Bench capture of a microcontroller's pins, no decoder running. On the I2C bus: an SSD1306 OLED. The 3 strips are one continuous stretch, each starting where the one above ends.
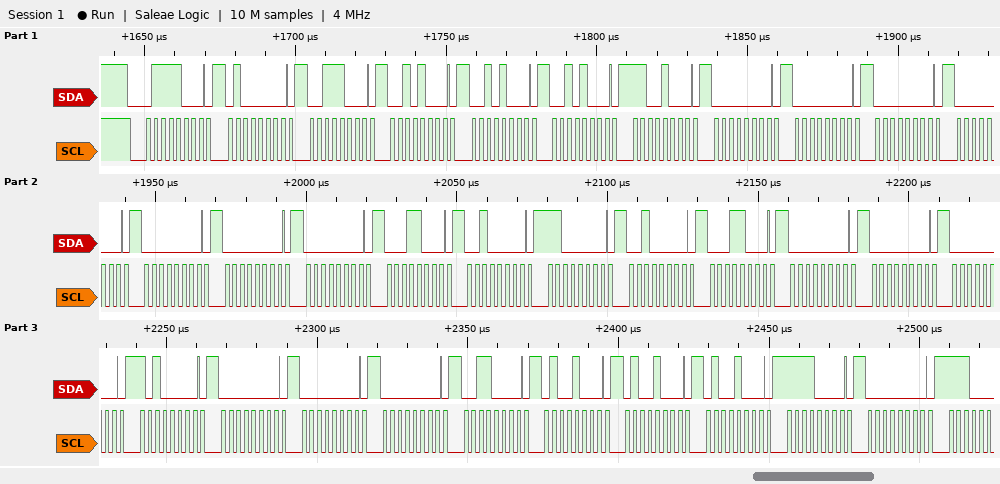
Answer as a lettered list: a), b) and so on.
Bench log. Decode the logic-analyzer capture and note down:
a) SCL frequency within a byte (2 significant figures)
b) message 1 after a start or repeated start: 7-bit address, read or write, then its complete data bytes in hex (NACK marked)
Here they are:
a) 400 kHz
b) 0x3C write: 40 38 28 28 28 C8 00 00 00 00 00 00 00 18 20 C0 20 18 00 00 00 A0 00 00 00 30 48 48 48 F0 00
